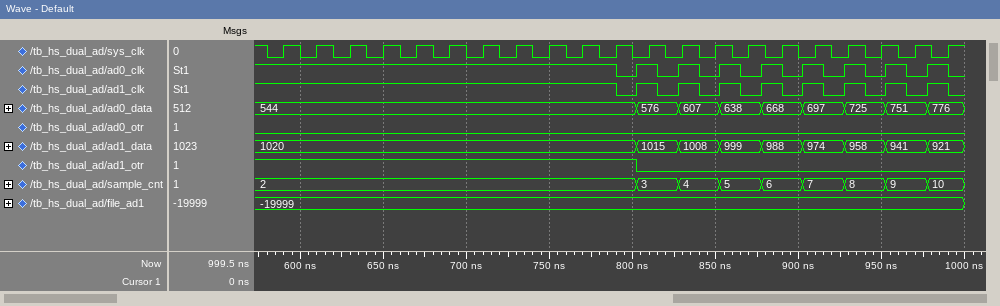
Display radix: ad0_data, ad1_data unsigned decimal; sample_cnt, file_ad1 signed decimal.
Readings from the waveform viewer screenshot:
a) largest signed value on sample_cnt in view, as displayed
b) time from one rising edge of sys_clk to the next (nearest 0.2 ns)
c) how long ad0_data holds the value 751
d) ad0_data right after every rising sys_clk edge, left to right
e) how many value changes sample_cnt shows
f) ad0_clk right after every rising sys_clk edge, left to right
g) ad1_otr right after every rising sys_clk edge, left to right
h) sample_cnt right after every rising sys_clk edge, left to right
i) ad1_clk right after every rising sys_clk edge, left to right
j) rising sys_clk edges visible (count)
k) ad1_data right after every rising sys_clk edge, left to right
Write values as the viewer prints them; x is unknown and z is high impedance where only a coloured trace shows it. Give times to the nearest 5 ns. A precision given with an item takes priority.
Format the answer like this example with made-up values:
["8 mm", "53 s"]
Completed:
["10", "20 ns", "25 ns", "544, 544, 544, 544, 544, 544, 544, 544, 544, 544, 544, 576, 607, 607, 638, 668, 697, 725, 725, 751, 776", "8", "1 1 1 1 1 1 1 1 1 1 0 1 1 0 0 0 1 1 0 0 0", "1 1 1 1 1 1 1 1 1 1 1 0 0 0 0 0 0 0 0 0 0", "2, 2, 2, 2, 2, 2, 2, 2, 2, 2, 2, 3, 4, 4, 5, 6, 7, 8, 8, 9, 10", "1 1 1 1 1 1 1 1 1 1 0 1 1 0 0 0 1 1 0 0 0", "21", "1020, 1020, 1020, 1020, 1020, 1020, 1020, 1020, 1020, 1020, 1020, 1015, 1008, 1008, 999, 988, 974, 958, 958, 941, 921"]
